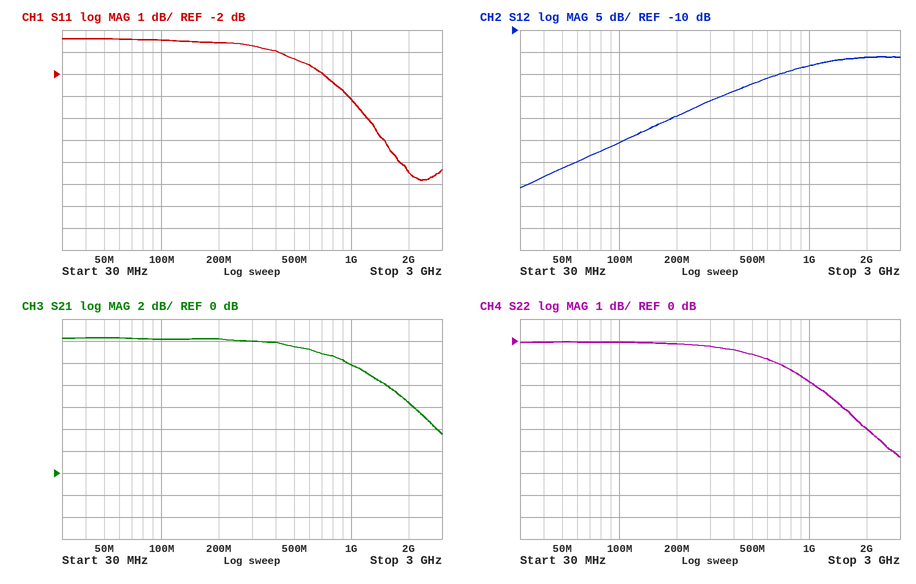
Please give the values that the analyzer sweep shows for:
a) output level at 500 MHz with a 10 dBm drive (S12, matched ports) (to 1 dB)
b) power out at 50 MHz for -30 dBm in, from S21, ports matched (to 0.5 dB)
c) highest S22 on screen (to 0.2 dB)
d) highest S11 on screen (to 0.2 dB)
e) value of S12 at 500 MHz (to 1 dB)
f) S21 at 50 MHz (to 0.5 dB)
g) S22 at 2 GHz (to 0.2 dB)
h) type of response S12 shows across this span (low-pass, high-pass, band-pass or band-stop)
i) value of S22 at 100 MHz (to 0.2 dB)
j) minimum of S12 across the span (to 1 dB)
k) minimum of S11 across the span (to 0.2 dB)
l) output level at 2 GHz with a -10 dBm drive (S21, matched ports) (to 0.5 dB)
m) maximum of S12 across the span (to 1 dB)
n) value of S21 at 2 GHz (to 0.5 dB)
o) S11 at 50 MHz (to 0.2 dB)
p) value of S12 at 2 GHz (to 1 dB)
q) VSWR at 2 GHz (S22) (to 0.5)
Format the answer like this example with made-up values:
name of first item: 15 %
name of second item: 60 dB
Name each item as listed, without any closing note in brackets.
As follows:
output level at 500 MHz with a 10 dBm drive (S12, matched ports): -12 dBm
power out at 50 MHz for -30 dBm in, from S21, ports matched: -17.5 dBm
highest S22 on screen: 0.0 dB
highest S11 on screen: -0.4 dB
value of S12 at 500 MHz: -22 dB
S21 at 50 MHz: 12.5 dB
S22 at 2 GHz: -4.0 dB
type of response S12 shows across this span: high-pass
value of S22 at 100 MHz: 0.0 dB
minimum of S12 across the span: -46 dB
minimum of S11 across the span: -6.8 dB
output level at 2 GHz with a -10 dBm drive (S21, matched ports): -3.5 dBm
maximum of S12 across the span: -16 dB
value of S21 at 2 GHz: 6.5 dB
S11 at 50 MHz: -0.4 dB
value of S12 at 2 GHz: -16 dB
VSWR at 2 GHz (S22): 4.5
